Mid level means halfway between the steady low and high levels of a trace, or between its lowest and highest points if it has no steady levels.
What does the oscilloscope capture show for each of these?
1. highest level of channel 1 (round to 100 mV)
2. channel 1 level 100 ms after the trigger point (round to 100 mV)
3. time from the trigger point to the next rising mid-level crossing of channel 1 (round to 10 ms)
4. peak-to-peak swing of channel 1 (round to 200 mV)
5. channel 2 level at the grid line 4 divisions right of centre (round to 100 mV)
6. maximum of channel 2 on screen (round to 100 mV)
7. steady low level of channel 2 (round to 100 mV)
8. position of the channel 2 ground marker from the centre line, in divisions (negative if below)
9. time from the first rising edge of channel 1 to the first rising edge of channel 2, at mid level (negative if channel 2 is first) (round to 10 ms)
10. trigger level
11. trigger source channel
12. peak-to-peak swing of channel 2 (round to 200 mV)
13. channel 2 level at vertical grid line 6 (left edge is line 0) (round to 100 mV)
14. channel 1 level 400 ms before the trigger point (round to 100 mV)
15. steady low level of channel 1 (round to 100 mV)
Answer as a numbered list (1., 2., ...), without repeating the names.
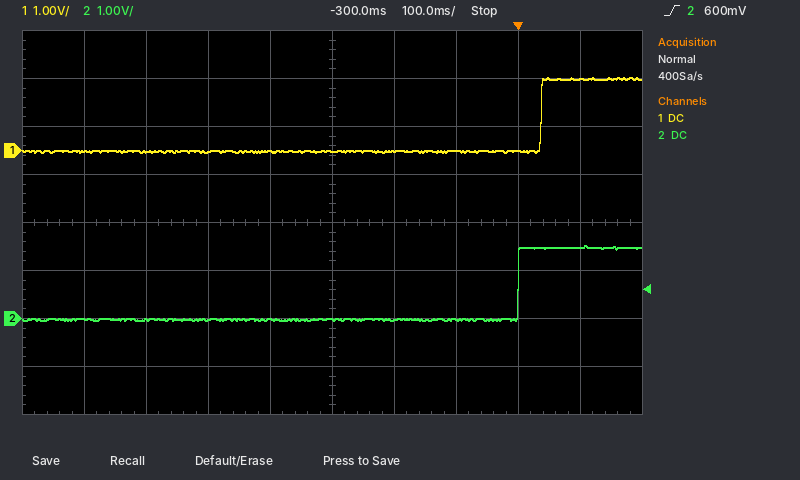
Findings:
1. 1.5 V
2. 1.5 V
3. 40 ms
4. 1.6 V
5. 1.5 V
6. 1.5 V
7. 0.0 V
8. -2.0 div
9. -40 ms
10. 600 mV
11. channel 2
12. 1.6 V
13. 0.0 V
14. 0.0 V
15. 0.0 V
